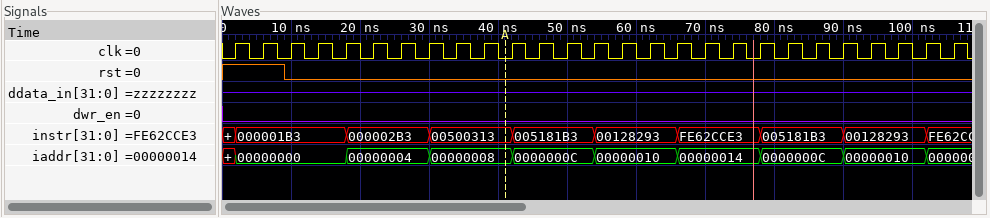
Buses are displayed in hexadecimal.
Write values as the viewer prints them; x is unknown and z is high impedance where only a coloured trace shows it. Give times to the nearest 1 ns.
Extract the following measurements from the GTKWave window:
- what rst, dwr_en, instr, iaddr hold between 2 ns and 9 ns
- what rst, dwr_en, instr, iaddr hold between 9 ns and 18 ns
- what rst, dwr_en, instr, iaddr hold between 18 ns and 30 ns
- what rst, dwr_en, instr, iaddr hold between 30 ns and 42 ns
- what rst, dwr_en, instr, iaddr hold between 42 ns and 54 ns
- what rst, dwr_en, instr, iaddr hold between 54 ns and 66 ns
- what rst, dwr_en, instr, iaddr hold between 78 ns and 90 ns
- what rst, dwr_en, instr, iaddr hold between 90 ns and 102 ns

rst=1, dwr_en=0, instr=000001B3, iaddr=00000000
rst=0, dwr_en=0, instr=000001B3, iaddr=00000000
rst=0, dwr_en=0, instr=000002B3, iaddr=00000004
rst=0, dwr_en=0, instr=00500313, iaddr=00000008
rst=0, dwr_en=0, instr=005181B3, iaddr=0000000C
rst=0, dwr_en=0, instr=00128293, iaddr=00000010
rst=0, dwr_en=0, instr=005181B3, iaddr=0000000C
rst=0, dwr_en=0, instr=00128293, iaddr=00000010
